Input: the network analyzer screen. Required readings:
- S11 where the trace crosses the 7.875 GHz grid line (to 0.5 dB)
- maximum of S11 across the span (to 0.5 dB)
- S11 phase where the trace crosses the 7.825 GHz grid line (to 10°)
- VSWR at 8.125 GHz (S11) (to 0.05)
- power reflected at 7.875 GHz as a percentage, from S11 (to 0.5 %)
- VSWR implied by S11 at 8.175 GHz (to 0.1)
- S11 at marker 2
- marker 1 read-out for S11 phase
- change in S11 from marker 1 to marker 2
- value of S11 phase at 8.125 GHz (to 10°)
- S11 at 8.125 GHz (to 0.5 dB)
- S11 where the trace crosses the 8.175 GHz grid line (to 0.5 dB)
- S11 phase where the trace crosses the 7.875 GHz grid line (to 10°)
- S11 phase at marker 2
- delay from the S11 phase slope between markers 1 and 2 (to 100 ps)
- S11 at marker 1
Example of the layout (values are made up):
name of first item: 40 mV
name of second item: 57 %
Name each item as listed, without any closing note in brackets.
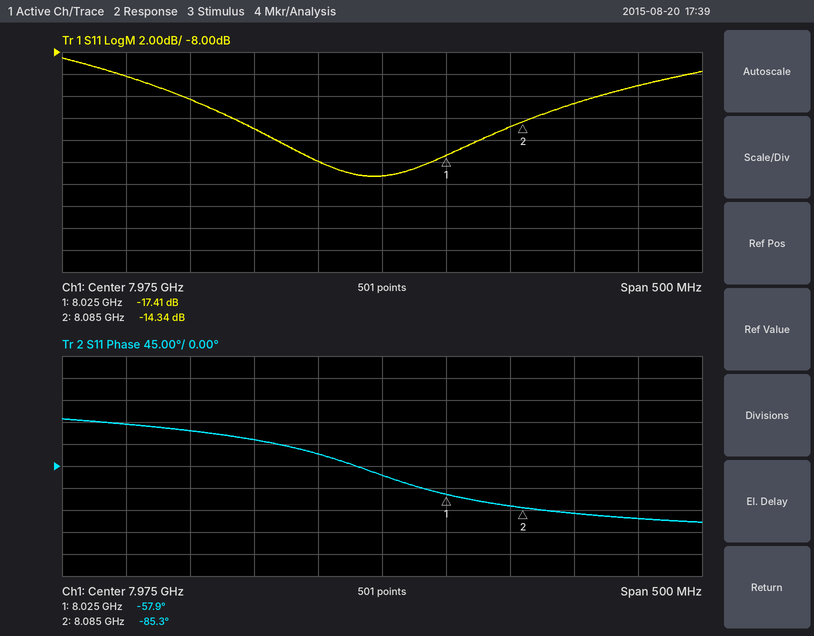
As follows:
S11 where the trace crosses the 7.875 GHz grid line: -15.0 dB
maximum of S11 across the span: -8.5 dB
S11 phase where the trace crosses the 7.825 GHz grid line: 70°
VSWR at 8.125 GHz (S11): 1.60
power reflected at 7.875 GHz as a percentage, from S11: 3.0 %
VSWR implied by S11 at 8.175 GHz: 1.8
S11 at marker 2: -14.34 dB
marker 1 read-out for S11 phase: -57.9°
change in S11 from marker 1 to marker 2: 3.07 dB
value of S11 phase at 8.125 GHz: -100°
S11 at 8.125 GHz: -12.5 dB
S11 where the trace crosses the 8.175 GHz grid line: -11.0 dB
S11 phase where the trace crosses the 7.875 GHz grid line: 50°
S11 phase at marker 2: -85.3°
delay from the S11 phase slope between markers 1 and 2: 1.3 ns
S11 at marker 1: -17.41 dB
